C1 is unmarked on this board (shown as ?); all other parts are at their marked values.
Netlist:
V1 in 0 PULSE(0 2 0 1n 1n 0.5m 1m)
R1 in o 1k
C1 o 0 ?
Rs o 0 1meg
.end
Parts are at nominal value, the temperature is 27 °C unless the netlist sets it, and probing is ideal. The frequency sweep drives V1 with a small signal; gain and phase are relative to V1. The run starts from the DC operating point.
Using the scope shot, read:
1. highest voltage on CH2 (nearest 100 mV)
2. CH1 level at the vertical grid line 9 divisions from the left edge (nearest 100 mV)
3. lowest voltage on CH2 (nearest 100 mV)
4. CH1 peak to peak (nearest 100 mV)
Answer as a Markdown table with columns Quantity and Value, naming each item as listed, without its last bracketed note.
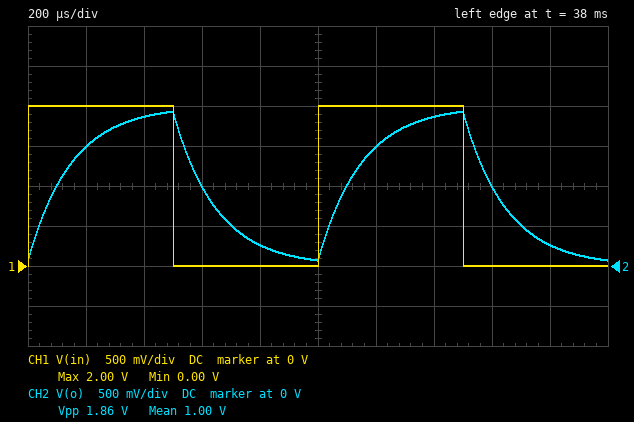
| Quantity | Value |
|---|---|
| highest voltage on CH2 | 1.9 V |
| CH1 level at the vertical grid line 9 divisions from the left edge | 0 V |
| lowest voltage on CH2 | 100 mV |
| CH1 peak to peak | 2.0 V |
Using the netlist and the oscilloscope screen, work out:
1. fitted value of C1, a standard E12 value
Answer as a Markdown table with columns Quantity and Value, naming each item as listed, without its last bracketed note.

| Quantity | Value |
|---|---|
| fitted value of C1, a standard E12 value | 150 nF |
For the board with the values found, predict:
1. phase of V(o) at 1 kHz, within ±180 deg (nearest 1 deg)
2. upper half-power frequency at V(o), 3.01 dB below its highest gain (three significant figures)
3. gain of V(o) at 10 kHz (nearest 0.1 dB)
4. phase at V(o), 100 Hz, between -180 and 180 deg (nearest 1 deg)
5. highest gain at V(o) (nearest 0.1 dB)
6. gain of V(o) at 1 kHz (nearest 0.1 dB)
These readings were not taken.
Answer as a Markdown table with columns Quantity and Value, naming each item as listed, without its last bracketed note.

| Quantity | Value |
|---|---|
| phase of V(o) at 1 kHz, within ±180 deg | -43 deg |
| upper half-power frequency at V(o), 3.01 dB below its highest gain | 1.06 kHz |
| gain of V(o) at 10 kHz | -19.5 dB |
| phase at V(o), 100 Hz, between -180 and 180 deg | -5 deg |
| highest gain at V(o) | 0 dB |
| gain of V(o) at 1 kHz | -2.8 dB |
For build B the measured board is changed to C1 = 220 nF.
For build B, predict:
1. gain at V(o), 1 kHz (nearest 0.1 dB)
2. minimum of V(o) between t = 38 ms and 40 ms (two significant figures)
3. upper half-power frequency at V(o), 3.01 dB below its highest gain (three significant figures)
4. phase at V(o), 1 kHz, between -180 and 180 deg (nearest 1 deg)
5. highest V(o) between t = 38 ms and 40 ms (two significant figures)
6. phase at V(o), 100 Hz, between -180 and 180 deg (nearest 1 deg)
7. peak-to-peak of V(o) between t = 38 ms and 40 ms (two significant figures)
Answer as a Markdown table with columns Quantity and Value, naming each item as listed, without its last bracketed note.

| Quantity | Value |
|---|---|
| gain at V(o), 1 kHz | -4.6 dB |
| minimum of V(o) between t = 38 ms and 40 ms | 190 mV |
| upper half-power frequency at V(o), 3.01 dB below its highest gain | 724 Hz |
| phase at V(o), 1 kHz, between -180 and 180 deg | -54 deg |
| highest V(o) between t = 38 ms and 40 ms | 1.8 V |
| phase at V(o), 100 Hz, between -180 and 180 deg | -8 deg |
| peak-to-peak of V(o) between t = 38 ms and 40 ms | 1.6 V |
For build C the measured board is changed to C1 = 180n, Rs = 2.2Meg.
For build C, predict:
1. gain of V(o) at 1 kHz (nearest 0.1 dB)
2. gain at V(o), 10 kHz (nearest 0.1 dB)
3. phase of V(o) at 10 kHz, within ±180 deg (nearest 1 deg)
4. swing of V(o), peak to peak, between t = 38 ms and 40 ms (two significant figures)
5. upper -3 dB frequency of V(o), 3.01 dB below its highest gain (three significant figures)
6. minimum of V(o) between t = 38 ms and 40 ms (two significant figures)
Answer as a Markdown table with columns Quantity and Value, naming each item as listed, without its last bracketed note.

| Quantity | Value |
|---|---|
| gain of V(o) at 1 kHz | -3.6 dB |
| gain at V(o), 10 kHz | -21.1 dB |
| phase of V(o) at 10 kHz, within ±180 deg | -85 deg |
| swing of V(o), peak to peak, between t = 38 ms and 40 ms | 1.8 V |
| upper -3 dB frequency of V(o), 3.01 dB below its highest gain | 885 Hz |
| minimum of V(o) between t = 38 ms and 40 ms | 120 mV |
